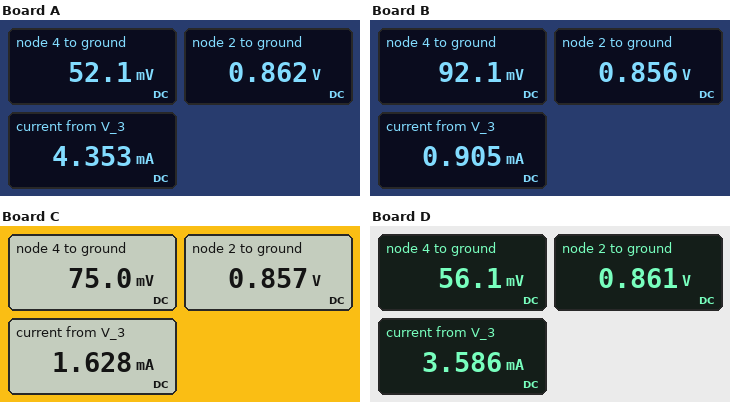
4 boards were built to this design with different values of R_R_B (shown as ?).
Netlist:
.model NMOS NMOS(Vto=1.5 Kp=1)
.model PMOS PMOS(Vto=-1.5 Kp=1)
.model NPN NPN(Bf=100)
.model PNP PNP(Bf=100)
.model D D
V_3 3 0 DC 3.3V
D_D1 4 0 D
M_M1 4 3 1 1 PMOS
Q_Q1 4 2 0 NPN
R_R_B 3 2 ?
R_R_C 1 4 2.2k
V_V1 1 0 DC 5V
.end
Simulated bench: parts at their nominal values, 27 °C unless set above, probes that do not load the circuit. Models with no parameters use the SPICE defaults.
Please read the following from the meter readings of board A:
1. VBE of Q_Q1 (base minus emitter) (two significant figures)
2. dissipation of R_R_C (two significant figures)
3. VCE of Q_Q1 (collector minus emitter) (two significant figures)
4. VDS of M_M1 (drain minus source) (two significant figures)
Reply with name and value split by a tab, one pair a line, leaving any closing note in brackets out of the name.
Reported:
VBE of Q_Q1 (base minus emitter)	860 mV
dissipation of R_R_C	11 mW
VCE of Q_Q1 (collector minus emitter)	52 mV
VDS of M_M1 (drain minus source)	-4.9 V
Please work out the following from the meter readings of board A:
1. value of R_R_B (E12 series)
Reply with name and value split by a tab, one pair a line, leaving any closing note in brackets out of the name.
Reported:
value of R_R_B	560 Ω
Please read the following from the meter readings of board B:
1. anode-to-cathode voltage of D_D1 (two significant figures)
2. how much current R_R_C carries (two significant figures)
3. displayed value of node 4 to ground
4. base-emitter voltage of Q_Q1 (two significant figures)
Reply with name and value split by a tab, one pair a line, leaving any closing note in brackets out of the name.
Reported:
anode-to-cathode voltage of D_D1	92 mV
how much current R_R_C carries	2.2 mA
displayed value of node 4 to ground	92.1 mV
base-emitter voltage of Q_Q1	860 mV
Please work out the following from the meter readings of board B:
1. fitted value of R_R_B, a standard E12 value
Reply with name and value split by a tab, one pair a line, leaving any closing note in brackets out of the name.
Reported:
fitted value of R_R_B, a standard E12 value	2.7 kΩ
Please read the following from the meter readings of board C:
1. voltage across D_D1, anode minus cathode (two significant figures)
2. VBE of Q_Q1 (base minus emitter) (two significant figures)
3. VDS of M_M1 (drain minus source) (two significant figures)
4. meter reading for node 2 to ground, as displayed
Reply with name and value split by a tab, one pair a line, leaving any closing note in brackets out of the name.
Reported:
voltage across D_D1, anode minus cathode	75 mV
VBE of Q_Q1 (base minus emitter)	860 mV
VDS of M_M1 (drain minus source)	-4.9 V
meter reading for node 2 to ground, as displayed	0.857 V
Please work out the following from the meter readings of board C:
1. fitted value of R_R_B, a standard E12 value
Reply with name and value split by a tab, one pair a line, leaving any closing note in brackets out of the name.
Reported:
fitted value of R_R_B, a standard E12 value	1.5 kΩ
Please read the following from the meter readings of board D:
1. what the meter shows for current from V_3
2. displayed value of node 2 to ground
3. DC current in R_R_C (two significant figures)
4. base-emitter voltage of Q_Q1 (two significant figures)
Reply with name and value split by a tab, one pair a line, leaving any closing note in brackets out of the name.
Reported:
what the meter shows for current from V_3	3.586 mA
displayed value of node 2 to ground	0.861 V
DC current in R_R_C	2.2 mA
base-emitter voltage of Q_Q1	860 mV
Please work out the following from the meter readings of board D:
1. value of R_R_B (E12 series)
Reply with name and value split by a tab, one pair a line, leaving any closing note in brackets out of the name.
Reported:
value of R_R_B	680 Ω
